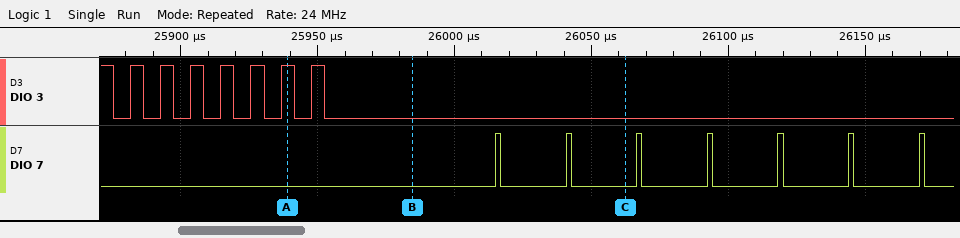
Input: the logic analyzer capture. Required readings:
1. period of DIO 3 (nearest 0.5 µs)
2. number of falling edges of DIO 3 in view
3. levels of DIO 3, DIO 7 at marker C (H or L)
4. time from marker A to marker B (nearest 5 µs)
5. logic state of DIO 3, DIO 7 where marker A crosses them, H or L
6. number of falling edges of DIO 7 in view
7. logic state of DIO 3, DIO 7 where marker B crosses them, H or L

11 µs
8
DIO 3=L, DIO 7=L
45 µs
DIO 3=H, DIO 7=L
7
DIO 3=L, DIO 7=L
